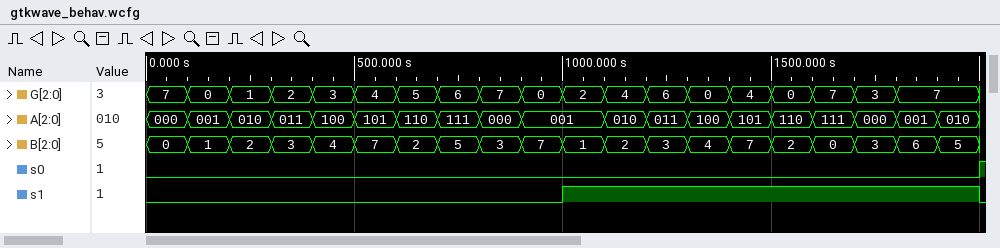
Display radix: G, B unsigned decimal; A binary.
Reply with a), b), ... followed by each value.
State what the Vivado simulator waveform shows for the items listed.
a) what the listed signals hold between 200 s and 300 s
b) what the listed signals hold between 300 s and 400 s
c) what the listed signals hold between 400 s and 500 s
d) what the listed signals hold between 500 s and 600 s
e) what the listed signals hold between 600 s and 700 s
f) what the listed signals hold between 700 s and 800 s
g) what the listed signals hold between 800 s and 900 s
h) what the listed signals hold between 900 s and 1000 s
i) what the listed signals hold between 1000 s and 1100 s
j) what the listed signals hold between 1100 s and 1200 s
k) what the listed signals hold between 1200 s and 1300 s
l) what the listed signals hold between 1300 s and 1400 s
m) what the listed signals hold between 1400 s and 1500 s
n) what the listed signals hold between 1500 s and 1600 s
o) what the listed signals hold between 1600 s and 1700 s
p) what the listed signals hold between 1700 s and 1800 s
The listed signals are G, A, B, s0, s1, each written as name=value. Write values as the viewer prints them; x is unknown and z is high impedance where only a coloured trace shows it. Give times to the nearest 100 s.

a) G=1, A=010, B=2, s0=0, s1=0
b) G=2, A=011, B=3, s0=0, s1=0
c) G=3, A=100, B=4, s0=0, s1=0
d) G=4, A=101, B=7, s0=0, s1=0
e) G=5, A=110, B=2, s0=0, s1=0
f) G=6, A=111, B=5, s0=0, s1=0
g) G=7, A=000, B=3, s0=0, s1=0
h) G=0, A=001, B=7, s0=0, s1=0
i) G=2, A=001, B=1, s0=0, s1=1
j) G=4, A=010, B=2, s0=0, s1=1
k) G=6, A=011, B=3, s0=0, s1=1
l) G=0, A=100, B=4, s0=0, s1=1
m) G=4, A=101, B=7, s0=0, s1=1
n) G=0, A=110, B=2, s0=0, s1=1
o) G=7, A=111, B=0, s0=0, s1=1
p) G=3, A=000, B=3, s0=0, s1=1
